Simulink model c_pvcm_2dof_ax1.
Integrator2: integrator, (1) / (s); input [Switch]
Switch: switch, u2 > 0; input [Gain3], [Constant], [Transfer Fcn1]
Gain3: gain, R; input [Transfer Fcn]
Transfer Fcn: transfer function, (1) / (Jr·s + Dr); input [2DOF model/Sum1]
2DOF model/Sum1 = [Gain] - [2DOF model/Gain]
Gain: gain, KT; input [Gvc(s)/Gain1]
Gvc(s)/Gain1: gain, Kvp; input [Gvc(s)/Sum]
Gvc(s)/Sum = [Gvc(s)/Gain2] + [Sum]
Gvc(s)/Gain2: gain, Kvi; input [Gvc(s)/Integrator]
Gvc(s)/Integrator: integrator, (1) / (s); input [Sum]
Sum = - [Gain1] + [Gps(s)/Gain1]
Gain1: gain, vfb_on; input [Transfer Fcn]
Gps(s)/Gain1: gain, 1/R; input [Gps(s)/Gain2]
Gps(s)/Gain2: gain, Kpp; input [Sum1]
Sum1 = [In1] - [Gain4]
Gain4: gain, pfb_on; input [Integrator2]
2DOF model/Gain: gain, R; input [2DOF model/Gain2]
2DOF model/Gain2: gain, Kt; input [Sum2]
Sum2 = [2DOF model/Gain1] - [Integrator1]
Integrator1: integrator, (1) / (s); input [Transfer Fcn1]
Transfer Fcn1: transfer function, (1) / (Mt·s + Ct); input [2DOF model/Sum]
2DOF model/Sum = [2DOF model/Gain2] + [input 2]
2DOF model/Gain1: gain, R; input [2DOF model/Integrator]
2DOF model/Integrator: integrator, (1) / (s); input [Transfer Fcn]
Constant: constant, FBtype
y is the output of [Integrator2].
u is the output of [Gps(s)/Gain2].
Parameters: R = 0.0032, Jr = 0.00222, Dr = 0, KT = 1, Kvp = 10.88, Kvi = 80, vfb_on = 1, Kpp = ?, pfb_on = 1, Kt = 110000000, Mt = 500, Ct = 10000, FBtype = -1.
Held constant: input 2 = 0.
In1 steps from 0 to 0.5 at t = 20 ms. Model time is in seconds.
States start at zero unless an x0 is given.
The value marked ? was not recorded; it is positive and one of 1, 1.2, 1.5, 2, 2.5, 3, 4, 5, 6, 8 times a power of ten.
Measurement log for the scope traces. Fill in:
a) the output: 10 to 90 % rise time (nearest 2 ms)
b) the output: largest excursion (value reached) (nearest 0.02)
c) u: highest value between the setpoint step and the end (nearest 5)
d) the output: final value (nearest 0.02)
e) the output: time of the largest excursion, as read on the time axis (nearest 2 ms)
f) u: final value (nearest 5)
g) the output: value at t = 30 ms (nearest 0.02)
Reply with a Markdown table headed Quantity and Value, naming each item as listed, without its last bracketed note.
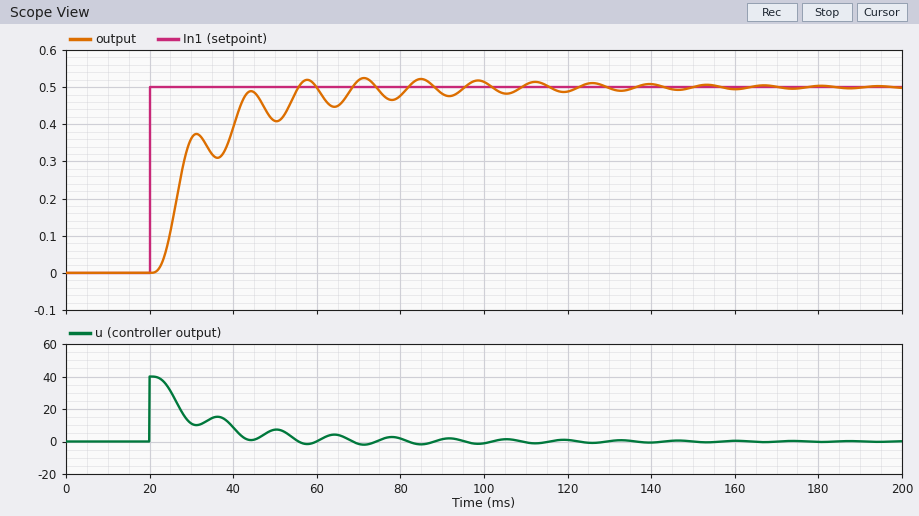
| Quantity | Value |
|---|---|
| the output: 10 to 90 % rise time | 18 ms |
| the output: largest excursion (value reached) | 0.52 |
| u: highest value between the setpoint step and the end | 40 |
| the output: final value | 0.50 |
| the output: time of the largest excursion, as read on the time axis | 72 ms |
| u: final value | 0 |
| the output: value at t = 30 ms | 0.36 |
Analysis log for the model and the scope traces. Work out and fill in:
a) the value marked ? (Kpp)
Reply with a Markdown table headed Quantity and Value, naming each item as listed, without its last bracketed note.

| Quantity | Value |
|---|---|
| the value marked ? | 80 |
